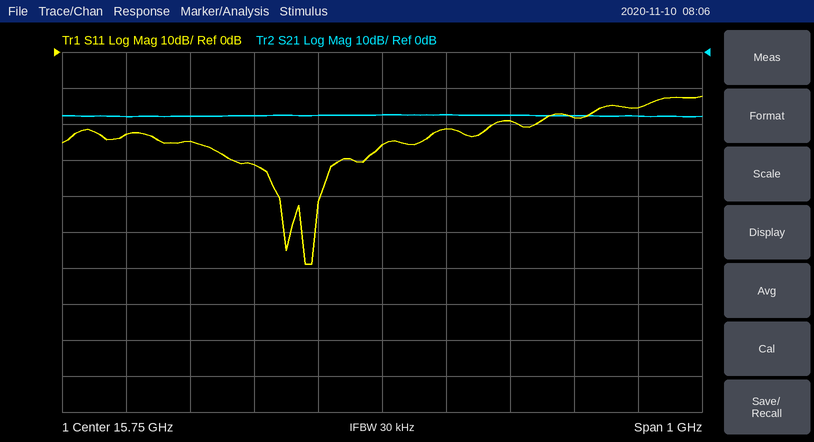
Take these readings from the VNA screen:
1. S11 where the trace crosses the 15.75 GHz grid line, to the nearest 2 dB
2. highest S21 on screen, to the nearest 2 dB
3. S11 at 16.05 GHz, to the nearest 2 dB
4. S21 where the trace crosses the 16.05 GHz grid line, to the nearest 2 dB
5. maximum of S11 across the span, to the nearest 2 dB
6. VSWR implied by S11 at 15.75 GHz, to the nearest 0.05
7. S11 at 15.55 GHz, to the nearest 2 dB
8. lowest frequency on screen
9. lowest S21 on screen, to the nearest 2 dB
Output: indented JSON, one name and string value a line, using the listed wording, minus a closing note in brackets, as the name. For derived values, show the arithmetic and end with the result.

{
  "S11 where the trace crosses the 15.75 GHz grid line, to the nearest 2 dB": "-26 dB",
  "highest S21 on screen, to the nearest 2 dB": "-18 dB",
  "S11 at 16.05 GHz, to the nearest 2 dB": "-18 dB",
  "S21 where the trace crosses the 16.05 GHz grid line, to the nearest 2 dB": "-18 dB",
  "maximum of S11 across the span, to the nearest 2 dB": "-12 dB",
  "VSWR implied by S11 at 15.75 GHz, to the nearest 0.05": "|Γ| = 10^(-26/20) = 0.0501; VSWR = (1 + 0.0501)/(1 − 0.0501) ≈ 1.11, so 1.10 to the nearest 0.05",
  "S11 at 15.55 GHz, to the nearest 2 dB": "-32 dB",
  "lowest frequency on screen": "15.25 GHz",
  "lowest S21 on screen, to the nearest 2 dB": "-18 dB"
}
